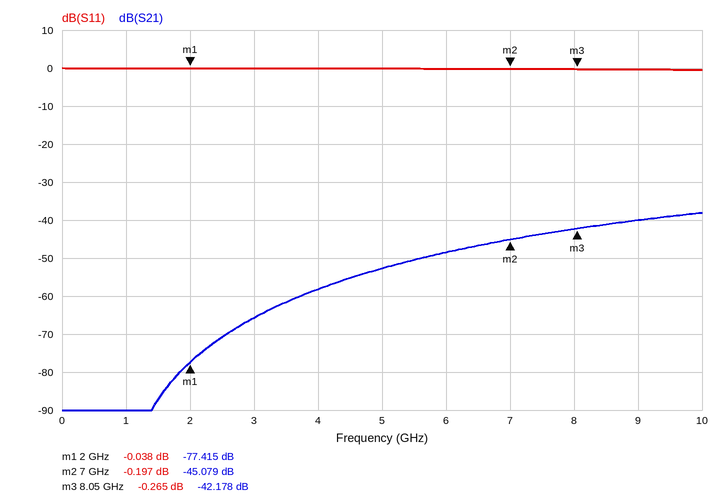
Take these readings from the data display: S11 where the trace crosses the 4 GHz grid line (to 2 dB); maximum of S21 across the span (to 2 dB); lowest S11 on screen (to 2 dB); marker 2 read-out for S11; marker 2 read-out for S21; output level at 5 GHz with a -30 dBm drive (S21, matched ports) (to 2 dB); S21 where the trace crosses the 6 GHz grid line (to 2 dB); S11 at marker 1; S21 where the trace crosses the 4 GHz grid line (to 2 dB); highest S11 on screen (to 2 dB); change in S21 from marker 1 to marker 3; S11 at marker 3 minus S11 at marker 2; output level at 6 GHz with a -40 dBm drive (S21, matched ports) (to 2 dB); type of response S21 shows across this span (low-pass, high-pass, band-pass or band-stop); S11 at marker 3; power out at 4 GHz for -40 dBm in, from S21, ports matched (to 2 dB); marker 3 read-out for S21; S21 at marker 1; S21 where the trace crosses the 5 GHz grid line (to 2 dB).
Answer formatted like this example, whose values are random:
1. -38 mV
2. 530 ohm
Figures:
1. 0 dB
2. -38 dB
3. 0 dB
4. -0.197 dB
5. -45.079 dB
6. -82 dBm
7. -48 dB
8. -0.038 dB
9. -58 dB
10. 0 dB
11. 35.237 dB
12. -0.068 dB
13. -88 dBm
14. high-pass
15. -0.265 dB
16. -98 dBm
17. -42.178 dB
18. -77.415 dB
19. -52 dB
